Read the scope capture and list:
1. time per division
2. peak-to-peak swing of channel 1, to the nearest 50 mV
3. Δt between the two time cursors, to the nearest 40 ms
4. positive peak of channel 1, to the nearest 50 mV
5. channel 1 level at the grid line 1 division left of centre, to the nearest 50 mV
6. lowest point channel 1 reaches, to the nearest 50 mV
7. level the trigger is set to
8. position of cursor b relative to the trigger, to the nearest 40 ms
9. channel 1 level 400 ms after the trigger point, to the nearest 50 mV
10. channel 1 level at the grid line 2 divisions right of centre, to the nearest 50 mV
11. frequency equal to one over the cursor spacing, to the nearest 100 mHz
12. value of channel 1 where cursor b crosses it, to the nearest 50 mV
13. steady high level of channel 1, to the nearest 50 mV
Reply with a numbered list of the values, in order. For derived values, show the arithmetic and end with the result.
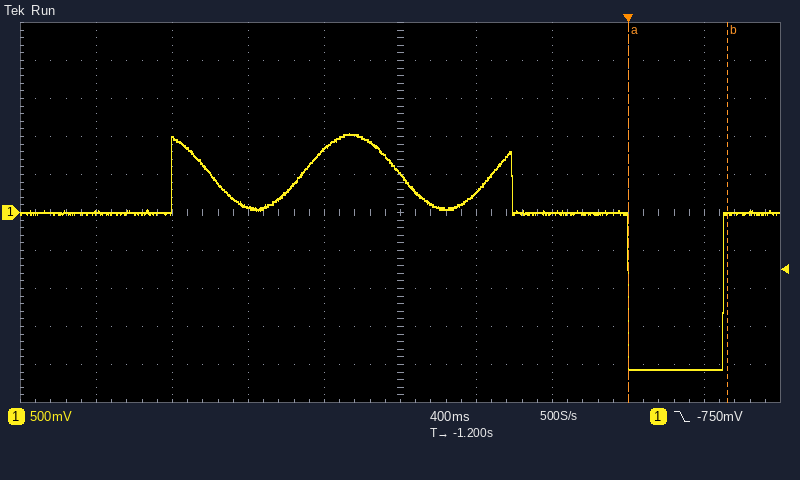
1. 400 ms
2. 1.05 V − (-2.05 V) = 3.10 V
3. 520 ms
4. 1.05 V
5. 850 mV
6. -2.05 V
7. -750 mV
8. +520 ms
9. -2.05 V
10. 0 mV
11. 1 / 520 ms ≈ 1.9 Hz
12. 0 mV
13. 0 mV
